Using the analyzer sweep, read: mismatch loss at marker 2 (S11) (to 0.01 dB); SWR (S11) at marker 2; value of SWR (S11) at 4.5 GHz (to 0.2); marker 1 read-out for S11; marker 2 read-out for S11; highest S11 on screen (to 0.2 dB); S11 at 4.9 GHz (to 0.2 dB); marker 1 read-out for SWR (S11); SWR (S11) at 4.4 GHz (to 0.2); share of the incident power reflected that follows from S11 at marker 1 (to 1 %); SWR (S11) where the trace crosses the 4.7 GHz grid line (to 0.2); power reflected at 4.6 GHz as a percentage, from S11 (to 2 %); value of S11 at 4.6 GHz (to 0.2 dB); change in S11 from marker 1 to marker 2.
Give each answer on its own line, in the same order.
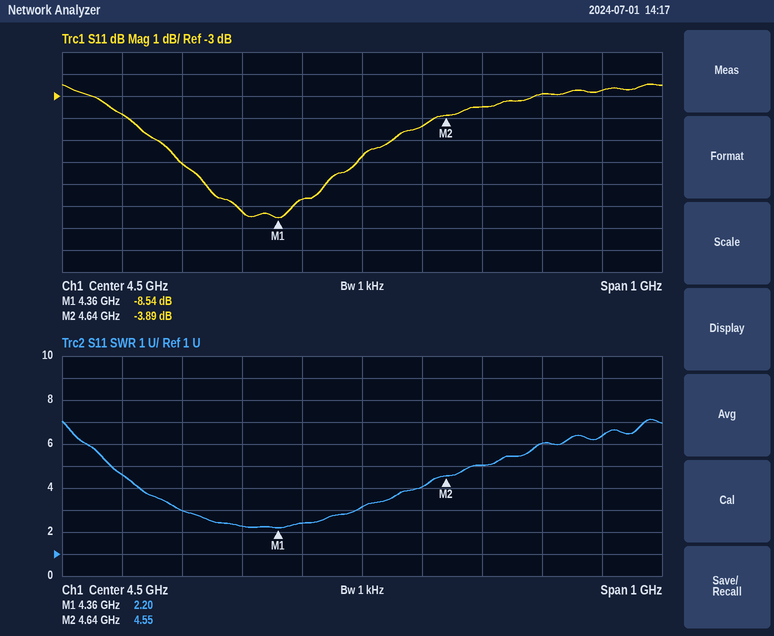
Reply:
2.28 dB
4.55
3.2
-8.54 dB
-3.89 dB
-2.4 dB
-2.8 dB
2.20
2.4
14 %
5.0
36 %
-4.4 dB
4.65 dB
